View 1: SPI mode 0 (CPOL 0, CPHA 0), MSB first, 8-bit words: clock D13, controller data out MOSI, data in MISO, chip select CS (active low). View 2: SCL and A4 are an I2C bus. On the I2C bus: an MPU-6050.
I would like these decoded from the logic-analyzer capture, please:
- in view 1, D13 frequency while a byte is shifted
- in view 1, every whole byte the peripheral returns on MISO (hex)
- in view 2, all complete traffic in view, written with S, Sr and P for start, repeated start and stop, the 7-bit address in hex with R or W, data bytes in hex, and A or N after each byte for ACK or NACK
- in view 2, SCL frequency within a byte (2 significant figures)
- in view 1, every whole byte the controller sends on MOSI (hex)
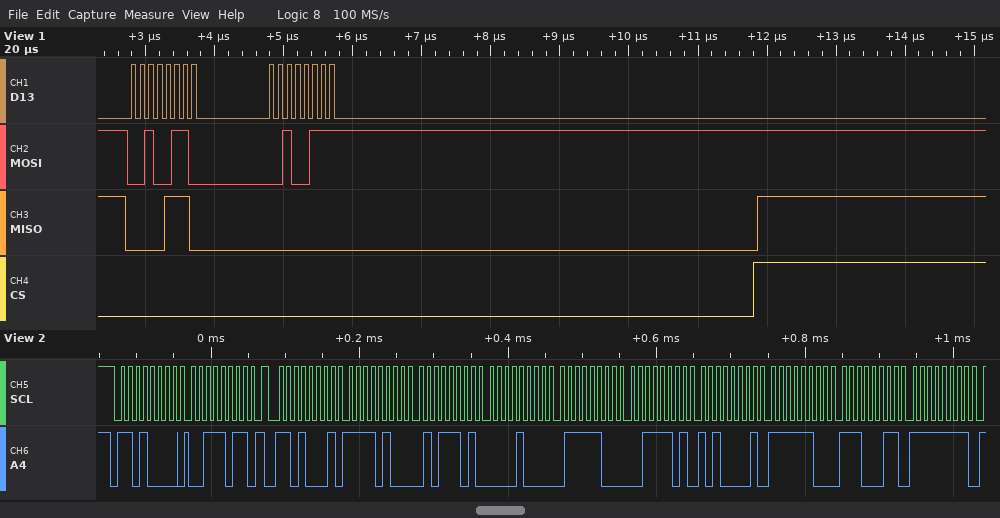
8 MHz
0E 00
S 68W A 3B A Sr 68R A F4 A 5D A 08 A 7C A 3D A A1 A FC A E3 A FF A
100 kHz
26 27
